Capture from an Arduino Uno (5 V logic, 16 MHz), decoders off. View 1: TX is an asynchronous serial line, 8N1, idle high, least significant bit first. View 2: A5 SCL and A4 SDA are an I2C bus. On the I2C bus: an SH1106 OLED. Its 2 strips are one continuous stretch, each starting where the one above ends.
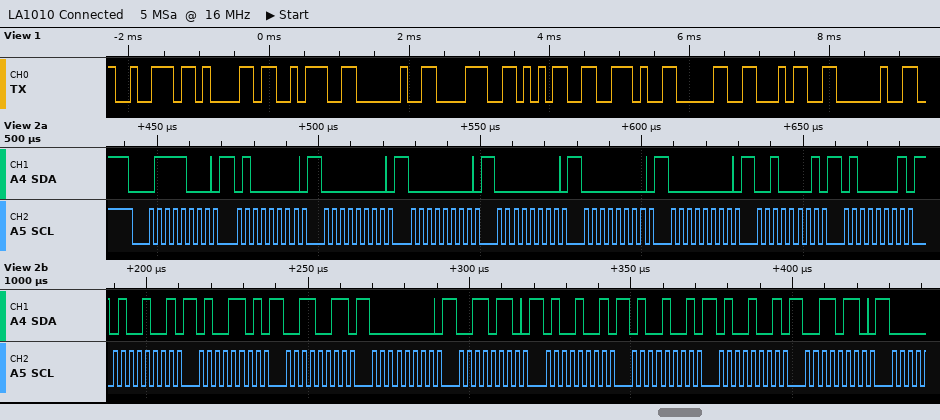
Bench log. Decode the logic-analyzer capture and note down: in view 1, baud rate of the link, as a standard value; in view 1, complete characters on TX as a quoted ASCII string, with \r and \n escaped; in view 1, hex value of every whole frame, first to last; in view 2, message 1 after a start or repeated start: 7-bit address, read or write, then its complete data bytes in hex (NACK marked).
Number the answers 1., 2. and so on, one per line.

1. 9600 baud
2. "ra: 85.04 "
3. 72 61 3A 20 38 35 2E 30 34 20
4. 0x3C write: 40 00 00 00 00 00 21 41 49 4D 33 00 36 49 49 49 36
